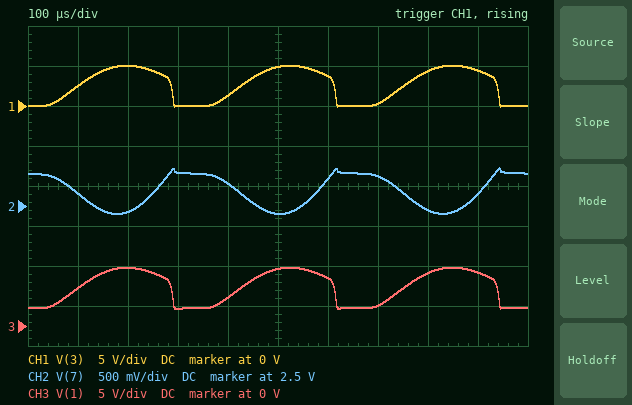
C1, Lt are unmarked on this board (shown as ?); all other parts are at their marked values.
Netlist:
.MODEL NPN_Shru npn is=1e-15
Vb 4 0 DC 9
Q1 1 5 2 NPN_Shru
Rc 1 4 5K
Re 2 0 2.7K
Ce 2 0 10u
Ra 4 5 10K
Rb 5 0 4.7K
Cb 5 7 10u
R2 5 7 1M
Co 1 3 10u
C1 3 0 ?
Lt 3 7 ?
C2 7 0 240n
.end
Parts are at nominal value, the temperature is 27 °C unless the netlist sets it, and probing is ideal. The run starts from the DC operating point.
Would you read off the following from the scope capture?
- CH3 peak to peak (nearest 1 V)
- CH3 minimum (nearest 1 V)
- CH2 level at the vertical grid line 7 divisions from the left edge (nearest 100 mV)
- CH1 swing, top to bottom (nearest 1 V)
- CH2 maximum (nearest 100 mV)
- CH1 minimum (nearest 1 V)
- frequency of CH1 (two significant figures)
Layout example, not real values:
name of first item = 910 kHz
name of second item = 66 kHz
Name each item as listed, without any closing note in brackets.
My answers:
CH3 peak to peak = 5 V
CH3 minimum = 2 V
CH2 level at the vertical grid line 7 divisions from the left edge = 2.9 V
CH1 swing, top to bottom = 5 V
CH2 maximum = 3.0 V
CH1 minimum = 0 V
frequency of CH1 = 3.1 kHz
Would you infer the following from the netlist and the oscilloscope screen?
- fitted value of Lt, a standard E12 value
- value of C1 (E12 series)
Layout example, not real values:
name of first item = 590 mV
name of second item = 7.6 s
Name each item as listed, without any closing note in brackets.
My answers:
fitted value of Lt, a standard E12 value = 100 mH
value of C1 = 47 nF
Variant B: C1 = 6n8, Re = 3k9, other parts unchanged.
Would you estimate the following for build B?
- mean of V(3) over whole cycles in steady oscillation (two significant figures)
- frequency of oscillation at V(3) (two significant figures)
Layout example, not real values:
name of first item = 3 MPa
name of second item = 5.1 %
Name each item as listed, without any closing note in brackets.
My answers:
mean of V(3) over whole cycles in steady oscillation = 2.8 V
frequency of oscillation at V(3) = 7.0 kHz
